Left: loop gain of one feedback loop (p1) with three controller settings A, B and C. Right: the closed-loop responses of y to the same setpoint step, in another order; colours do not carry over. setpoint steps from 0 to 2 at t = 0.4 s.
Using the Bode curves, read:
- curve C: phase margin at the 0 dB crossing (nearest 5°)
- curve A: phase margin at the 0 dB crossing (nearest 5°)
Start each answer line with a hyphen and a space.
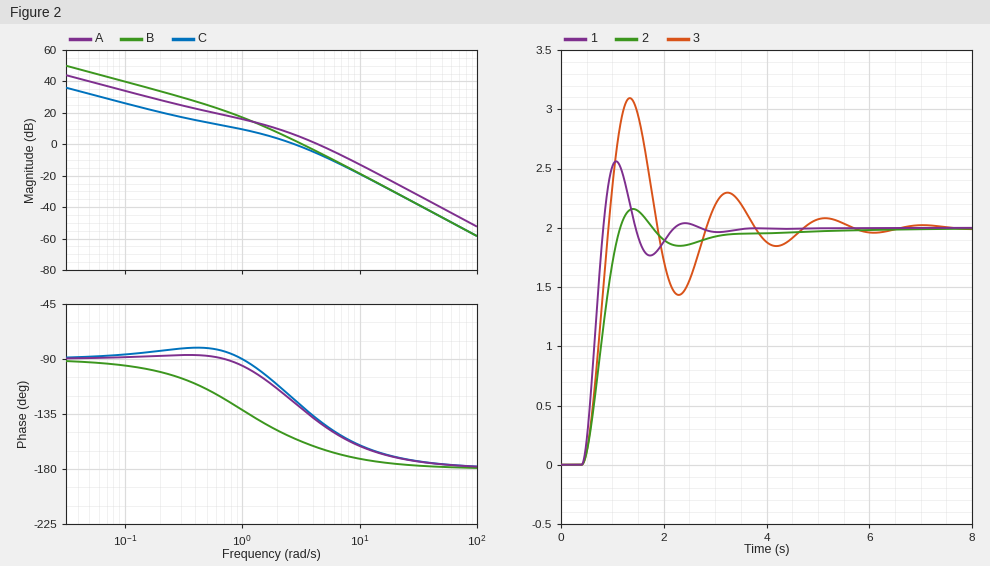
- 55°
- 40°
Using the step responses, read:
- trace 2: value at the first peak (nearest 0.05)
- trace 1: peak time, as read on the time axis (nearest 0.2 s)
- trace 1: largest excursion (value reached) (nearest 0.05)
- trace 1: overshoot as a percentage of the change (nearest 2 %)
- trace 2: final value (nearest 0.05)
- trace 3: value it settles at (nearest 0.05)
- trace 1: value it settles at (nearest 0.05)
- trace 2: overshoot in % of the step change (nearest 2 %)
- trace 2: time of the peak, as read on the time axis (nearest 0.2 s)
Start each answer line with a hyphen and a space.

- 2.15
- 1.0 s
- 2.55
- 28 %
- 2.00
- 2.00
- 2.00
- 8 %
- 1.4 s
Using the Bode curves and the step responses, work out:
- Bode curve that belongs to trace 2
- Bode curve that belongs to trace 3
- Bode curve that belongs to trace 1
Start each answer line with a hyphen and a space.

- C
- B
- A
